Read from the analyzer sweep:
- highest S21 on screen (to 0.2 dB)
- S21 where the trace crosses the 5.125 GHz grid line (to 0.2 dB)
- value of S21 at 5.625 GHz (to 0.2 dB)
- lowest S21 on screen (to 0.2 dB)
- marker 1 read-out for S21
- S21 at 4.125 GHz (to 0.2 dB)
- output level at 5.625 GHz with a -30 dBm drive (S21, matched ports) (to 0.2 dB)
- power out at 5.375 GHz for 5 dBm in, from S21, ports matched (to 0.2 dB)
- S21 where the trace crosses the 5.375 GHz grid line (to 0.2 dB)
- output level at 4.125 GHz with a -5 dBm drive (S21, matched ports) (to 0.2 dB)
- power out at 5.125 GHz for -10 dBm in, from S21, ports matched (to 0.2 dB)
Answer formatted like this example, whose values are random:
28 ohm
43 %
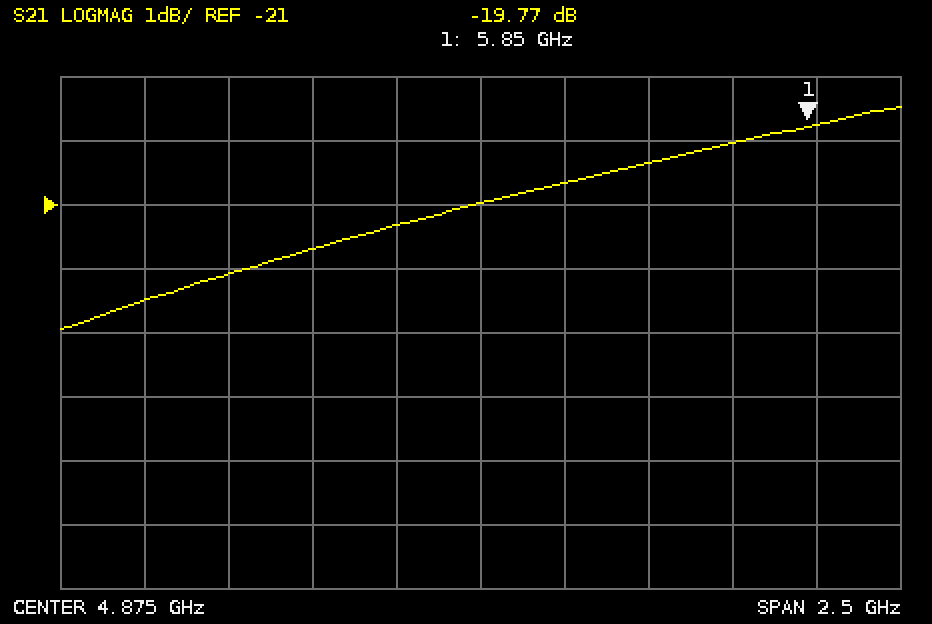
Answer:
-19.4 dB
-20.6 dB
-20.0 dB
-23.0 dB
-19.77 dB
-22.0 dB
-50.0 dBm
-15.4 dBm
-20.4 dB
-27.0 dBm
-30.6 dBm
